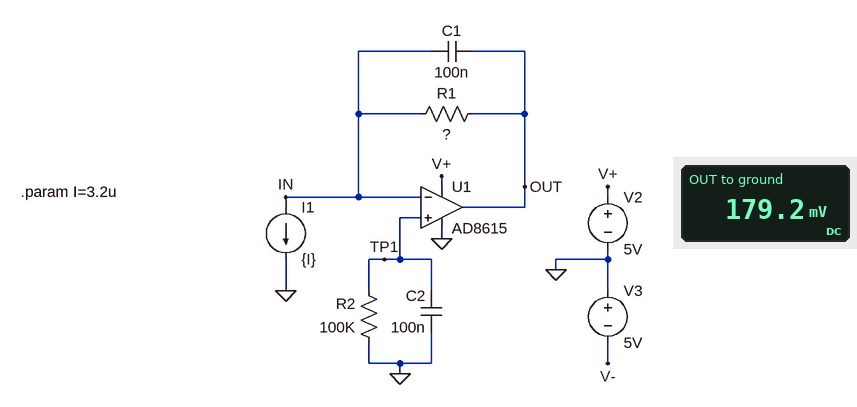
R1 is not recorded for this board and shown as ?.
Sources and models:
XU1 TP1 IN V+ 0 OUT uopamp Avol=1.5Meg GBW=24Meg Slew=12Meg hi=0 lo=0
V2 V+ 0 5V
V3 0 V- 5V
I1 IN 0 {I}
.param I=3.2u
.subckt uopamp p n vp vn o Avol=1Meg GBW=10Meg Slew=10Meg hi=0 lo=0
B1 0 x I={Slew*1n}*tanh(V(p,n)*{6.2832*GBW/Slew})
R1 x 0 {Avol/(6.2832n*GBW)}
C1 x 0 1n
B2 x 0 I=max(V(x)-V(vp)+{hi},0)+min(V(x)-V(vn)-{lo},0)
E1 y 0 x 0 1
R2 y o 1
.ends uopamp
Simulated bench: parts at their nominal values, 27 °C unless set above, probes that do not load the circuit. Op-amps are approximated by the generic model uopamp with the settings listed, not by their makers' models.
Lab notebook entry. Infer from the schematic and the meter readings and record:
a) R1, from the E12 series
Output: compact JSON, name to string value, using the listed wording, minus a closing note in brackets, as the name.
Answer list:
{"R1, from the E12 series": "56 kΩ"}
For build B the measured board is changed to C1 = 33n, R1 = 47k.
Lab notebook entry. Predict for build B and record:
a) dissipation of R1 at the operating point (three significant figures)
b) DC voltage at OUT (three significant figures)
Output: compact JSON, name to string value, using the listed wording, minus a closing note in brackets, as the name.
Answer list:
{"dissipation of R1 at the operating point": "481 nW", "DC voltage at OUT": "150 mV"}
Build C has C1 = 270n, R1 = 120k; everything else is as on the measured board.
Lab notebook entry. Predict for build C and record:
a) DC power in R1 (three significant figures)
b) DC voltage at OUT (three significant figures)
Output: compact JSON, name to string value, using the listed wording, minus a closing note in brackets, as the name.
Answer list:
{"DC power in R1": "1.23 µW", "DC voltage at OUT": "384 mV"}
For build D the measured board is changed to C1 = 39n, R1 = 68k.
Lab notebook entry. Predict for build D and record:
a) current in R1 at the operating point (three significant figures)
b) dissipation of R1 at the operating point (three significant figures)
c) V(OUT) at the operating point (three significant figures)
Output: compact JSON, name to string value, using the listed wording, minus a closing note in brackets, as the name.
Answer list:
{"current in R1 at the operating point": "3.20 µA", "dissipation of R1 at the operating point": "696 nW", "V(OUT) at the operating point": "218 mV"}
